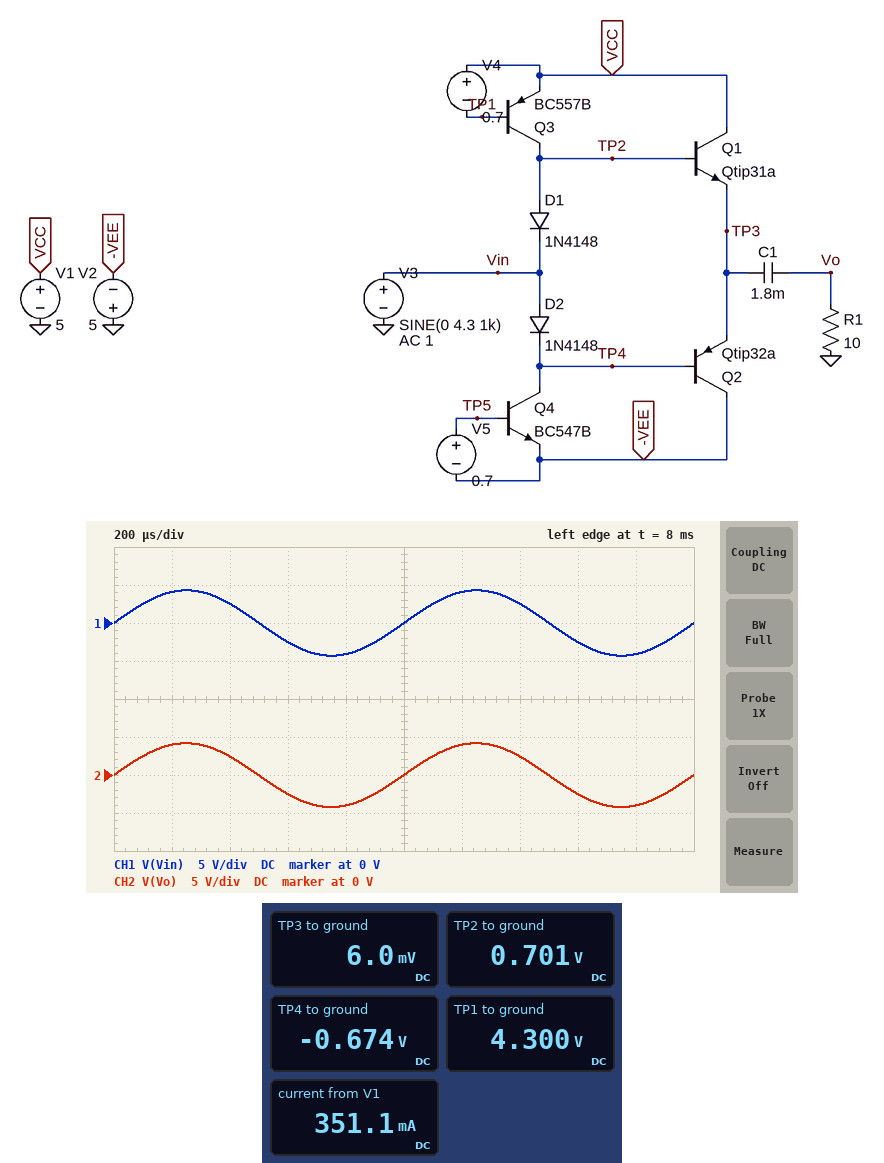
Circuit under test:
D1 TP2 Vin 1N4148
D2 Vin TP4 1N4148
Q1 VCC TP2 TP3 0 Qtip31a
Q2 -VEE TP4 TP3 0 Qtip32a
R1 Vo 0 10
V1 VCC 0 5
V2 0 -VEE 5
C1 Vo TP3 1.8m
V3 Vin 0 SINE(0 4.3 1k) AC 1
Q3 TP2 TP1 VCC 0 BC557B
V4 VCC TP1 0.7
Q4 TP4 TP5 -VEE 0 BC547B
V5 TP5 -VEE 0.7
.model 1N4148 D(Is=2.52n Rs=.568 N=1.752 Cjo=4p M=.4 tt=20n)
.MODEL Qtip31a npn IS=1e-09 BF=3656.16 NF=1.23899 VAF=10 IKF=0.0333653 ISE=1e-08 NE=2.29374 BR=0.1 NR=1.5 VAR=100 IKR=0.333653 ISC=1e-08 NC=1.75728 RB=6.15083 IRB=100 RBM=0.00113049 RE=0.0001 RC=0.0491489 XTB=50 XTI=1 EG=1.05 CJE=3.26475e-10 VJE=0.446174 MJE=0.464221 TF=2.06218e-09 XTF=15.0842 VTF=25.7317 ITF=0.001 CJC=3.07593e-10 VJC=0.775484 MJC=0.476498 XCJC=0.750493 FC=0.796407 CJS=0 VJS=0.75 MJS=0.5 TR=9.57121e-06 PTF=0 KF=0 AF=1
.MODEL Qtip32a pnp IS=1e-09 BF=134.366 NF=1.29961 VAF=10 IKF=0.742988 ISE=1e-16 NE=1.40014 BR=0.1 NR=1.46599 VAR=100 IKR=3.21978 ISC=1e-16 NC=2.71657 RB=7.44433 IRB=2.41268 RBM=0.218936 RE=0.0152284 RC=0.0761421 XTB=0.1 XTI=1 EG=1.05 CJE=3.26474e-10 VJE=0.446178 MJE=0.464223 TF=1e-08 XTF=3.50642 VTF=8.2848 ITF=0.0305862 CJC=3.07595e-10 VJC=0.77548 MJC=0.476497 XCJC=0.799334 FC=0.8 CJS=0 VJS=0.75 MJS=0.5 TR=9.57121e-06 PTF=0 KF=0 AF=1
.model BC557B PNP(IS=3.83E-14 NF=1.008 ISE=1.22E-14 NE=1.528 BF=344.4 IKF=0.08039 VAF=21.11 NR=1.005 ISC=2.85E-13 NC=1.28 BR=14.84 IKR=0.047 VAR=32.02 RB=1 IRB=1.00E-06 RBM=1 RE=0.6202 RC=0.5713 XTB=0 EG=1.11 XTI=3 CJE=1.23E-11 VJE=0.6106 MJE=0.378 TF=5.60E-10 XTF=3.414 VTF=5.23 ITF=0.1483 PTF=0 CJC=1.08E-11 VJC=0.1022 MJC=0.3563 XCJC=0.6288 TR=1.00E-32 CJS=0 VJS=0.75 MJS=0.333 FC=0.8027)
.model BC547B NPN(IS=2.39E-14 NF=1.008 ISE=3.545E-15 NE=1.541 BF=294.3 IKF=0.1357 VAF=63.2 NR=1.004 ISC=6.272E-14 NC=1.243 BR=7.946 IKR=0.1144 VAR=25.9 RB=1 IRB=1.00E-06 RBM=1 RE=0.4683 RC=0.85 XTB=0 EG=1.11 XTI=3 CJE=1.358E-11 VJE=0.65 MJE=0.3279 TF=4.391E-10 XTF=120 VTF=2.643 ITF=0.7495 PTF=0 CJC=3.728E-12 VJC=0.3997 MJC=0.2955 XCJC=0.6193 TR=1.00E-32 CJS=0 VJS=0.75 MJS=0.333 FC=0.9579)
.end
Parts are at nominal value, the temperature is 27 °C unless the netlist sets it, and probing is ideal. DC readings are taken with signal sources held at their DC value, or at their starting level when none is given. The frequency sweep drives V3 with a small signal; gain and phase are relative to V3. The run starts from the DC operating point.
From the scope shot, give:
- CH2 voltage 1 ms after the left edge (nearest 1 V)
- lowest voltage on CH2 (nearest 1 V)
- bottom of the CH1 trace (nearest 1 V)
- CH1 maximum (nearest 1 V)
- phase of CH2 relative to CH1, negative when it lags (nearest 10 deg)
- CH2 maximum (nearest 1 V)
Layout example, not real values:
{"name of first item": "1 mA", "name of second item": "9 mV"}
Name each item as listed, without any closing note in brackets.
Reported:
{"CH2 voltage 1 ms after the left edge": "0 V", "lowest voltage on CH2": "-4 V", "bottom of the CH1 trace": "-4 V", "CH1 maximum": "4 V", "phase of CH2 relative to CH1, negative when it lags": "0 deg", "CH2 maximum": "4 V"}
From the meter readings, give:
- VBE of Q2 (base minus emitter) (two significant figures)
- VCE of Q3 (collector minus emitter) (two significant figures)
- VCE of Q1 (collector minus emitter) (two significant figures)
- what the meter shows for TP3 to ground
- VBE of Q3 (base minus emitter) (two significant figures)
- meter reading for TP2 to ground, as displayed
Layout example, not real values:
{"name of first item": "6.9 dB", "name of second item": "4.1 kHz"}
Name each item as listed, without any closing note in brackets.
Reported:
{"VBE of Q2 (base minus emitter)": "-680 mV", "VCE of Q3 (collector minus emitter)": "-4.3 V", "VCE of Q1 (collector minus emitter)": "5.0 V", "what the meter shows for TP3 to ground": "6.0 mV", "VBE of Q3 (base minus emitter)": "-700 mV", "meter reading for TP2 to ground, as displayed": "0.701 V"}
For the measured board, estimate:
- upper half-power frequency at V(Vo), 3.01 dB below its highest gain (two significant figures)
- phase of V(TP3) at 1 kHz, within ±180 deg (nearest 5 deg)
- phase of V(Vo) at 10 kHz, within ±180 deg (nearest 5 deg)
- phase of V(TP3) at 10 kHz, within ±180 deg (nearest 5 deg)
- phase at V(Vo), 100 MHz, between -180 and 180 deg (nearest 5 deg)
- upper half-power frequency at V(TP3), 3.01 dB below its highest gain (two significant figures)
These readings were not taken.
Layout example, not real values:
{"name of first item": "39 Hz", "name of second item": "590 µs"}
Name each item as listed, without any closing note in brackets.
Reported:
{"upper half-power frequency at V(Vo), 3.01 dB below its highest gain": "4.4 MHz", "phase of V(TP3) at 1 kHz, within ±180 deg": "0 deg", "phase of V(Vo) at 10 kHz, within ±180 deg": "0 deg", "phase of V(TP3) at 10 kHz, within ±180 deg": "0 deg", "phase at V(Vo), 100 MHz, between -180 and 180 deg": "-15 deg", "upper half-power frequency at V(TP3), 3.01 dB below its highest gain": "4.2 MHz"}
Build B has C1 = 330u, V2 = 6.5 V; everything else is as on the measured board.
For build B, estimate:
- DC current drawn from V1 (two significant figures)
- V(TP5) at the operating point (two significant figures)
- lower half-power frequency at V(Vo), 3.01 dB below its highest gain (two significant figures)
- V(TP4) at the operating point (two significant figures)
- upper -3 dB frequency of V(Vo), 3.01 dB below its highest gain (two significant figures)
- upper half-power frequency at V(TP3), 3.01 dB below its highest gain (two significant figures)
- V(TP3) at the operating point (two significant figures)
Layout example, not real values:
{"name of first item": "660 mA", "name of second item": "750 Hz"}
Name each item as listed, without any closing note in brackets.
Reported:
{"DC current drawn from V1": "370 mA", "V(TP5) at the operating point": "-5.8 V", "lower half-power frequency at V(Vo), 3.01 dB below its highest gain": "48 Hz", "V(TP4) at the operating point": "-680 mV", "upper -3 dB frequency of V(Vo), 3.01 dB below its highest gain": "4.6 MHz", "upper half-power frequency at V(TP3), 3.01 dB below its highest gain": "4.4 MHz", "V(TP3) at the operating point": "1.4 mV"}
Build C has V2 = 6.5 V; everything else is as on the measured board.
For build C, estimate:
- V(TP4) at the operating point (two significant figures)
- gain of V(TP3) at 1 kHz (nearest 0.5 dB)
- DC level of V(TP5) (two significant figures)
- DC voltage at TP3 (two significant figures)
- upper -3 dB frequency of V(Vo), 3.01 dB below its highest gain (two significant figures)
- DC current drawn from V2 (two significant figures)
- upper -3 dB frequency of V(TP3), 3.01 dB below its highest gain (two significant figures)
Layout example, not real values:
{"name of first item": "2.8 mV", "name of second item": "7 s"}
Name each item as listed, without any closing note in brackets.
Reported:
{"V(TP4) at the operating point": "-680 mV", "gain of V(TP3) at 1 kHz": "0 dB", "DC level of V(TP5)": "-5.8 V", "DC voltage at TP3": "1.4 mV", "upper -3 dB frequency of V(Vo), 3.01 dB below its highest gain": "4.6 MHz", "DC current drawn from V2": "370 mA", "upper -3 dB frequency of V(TP3), 3.01 dB below its highest gain": "4.4 MHz"}
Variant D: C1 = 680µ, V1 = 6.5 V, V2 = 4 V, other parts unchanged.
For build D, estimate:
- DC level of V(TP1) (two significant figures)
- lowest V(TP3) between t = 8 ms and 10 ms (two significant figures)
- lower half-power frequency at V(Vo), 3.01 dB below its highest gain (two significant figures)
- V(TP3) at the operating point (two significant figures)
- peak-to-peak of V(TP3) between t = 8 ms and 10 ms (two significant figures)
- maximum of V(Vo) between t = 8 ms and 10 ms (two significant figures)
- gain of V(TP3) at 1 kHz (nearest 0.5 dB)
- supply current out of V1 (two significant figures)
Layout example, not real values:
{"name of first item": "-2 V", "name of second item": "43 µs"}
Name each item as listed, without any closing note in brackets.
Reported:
{"DC level of V(TP1)": "5.8 V", "lowest V(TP3) between t = 8 ms and 10 ms": "-3.3 V", "lower half-power frequency at V(Vo), 3.01 dB below its highest gain": "23 Hz", "V(TP3) at the operating point": "15 mV", "peak-to-peak of V(TP3) between t = 8 ms and 10 ms": "7.5 V", "maximum of V(Vo) between t = 8 ms and 10 ms": "4.1 V", "gain of V(TP3) at 1 kHz": "0 dB", "supply current out of V1": "360 mA"}
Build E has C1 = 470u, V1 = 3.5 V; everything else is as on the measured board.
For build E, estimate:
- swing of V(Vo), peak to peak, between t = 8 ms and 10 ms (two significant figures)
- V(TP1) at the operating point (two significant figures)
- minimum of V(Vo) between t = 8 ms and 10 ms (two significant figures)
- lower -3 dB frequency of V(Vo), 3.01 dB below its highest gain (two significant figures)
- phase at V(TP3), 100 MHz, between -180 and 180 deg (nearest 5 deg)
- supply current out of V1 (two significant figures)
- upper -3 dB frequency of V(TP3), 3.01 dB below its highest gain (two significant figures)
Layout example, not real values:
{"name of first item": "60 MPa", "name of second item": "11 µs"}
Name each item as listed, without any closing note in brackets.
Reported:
{"swing of V(Vo), peak to peak, between t = 8 ms and 10 ms": "7.0 V", "V(TP1) at the operating point": "2.8 V", "minimum of V(Vo) between t = 8 ms and 10 ms": "-4.0 V", "lower -3 dB frequency of V(Vo), 3.01 dB below its highest gain": "33 Hz", "phase at V(TP3), 100 MHz, between -180 and 180 deg": "-20 deg", "supply current out of V1": "330 mA", "upper -3 dB frequency of V(TP3), 3.01 dB below its highest gain": "4.1 MHz"}
